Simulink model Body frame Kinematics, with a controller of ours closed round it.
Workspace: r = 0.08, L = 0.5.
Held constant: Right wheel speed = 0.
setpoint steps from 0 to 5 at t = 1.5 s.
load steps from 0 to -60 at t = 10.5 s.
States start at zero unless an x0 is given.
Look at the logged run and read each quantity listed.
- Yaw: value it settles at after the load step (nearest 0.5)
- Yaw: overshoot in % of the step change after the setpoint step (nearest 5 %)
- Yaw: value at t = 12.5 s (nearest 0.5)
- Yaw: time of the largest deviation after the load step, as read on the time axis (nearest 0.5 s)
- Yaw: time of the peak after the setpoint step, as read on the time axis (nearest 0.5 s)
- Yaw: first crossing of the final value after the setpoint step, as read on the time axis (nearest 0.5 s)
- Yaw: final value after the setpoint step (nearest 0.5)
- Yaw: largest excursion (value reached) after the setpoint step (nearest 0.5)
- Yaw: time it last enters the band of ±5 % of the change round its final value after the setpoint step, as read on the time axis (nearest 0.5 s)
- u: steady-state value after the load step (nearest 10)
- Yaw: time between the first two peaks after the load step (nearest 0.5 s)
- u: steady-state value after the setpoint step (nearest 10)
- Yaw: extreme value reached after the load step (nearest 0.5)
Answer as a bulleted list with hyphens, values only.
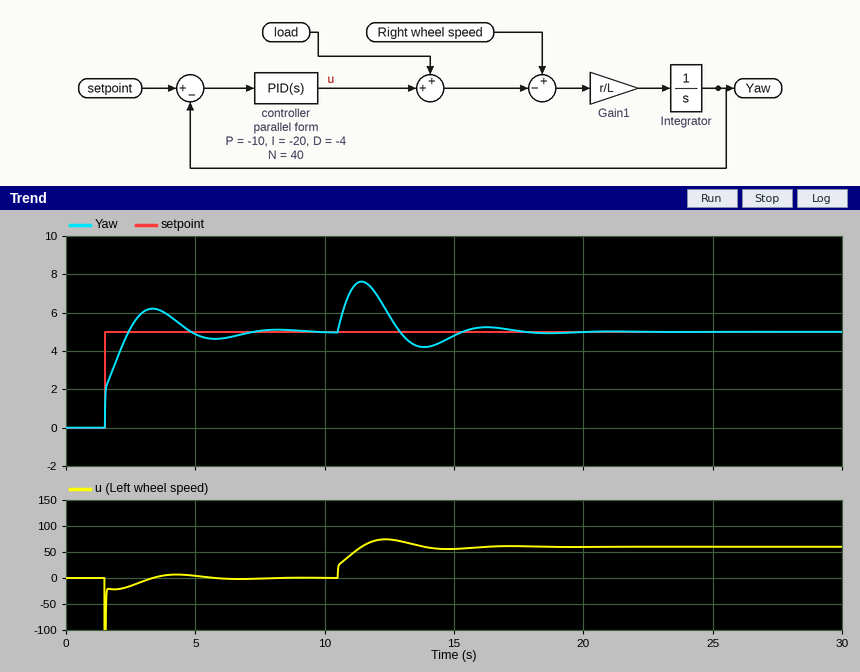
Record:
- 5.0
- 25 %
- 6.0
- 11.5 s
- 3.5 s
- 2.5 s
- 5.0
- 6.0
- 6.5 s
- 60
- 5.0 s
- 0
- 7.5
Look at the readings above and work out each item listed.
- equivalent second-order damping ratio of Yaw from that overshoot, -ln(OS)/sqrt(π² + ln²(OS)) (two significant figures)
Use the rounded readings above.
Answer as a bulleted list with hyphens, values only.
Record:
- 0.40
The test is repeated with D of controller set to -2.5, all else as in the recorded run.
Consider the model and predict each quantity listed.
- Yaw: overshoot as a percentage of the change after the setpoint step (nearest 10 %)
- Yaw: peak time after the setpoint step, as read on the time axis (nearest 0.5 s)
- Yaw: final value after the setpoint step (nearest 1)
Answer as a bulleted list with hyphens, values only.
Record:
- 30 %
- 3.0 s
- 5
